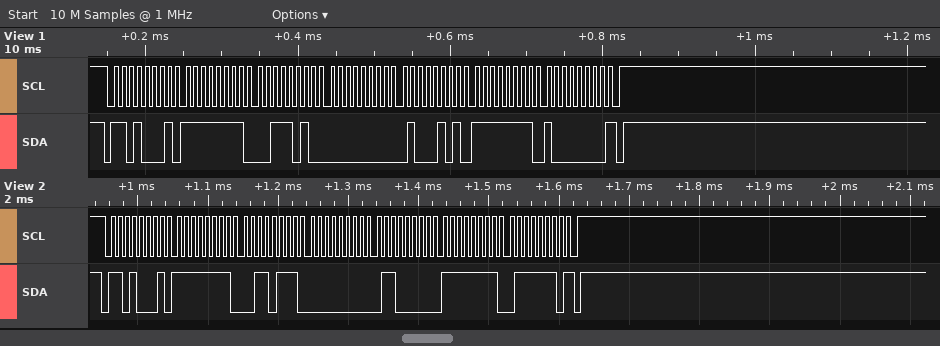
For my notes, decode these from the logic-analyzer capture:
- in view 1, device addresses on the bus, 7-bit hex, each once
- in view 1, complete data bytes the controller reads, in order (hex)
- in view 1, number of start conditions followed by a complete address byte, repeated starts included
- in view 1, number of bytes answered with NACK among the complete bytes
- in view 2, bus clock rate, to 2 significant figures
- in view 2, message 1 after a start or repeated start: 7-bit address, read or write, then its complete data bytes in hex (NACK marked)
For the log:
0x68
FF 3A 00 45 FF 80
1
1
100 kHz
0x68 read: FF 37 00 60 FF 7E NACK
